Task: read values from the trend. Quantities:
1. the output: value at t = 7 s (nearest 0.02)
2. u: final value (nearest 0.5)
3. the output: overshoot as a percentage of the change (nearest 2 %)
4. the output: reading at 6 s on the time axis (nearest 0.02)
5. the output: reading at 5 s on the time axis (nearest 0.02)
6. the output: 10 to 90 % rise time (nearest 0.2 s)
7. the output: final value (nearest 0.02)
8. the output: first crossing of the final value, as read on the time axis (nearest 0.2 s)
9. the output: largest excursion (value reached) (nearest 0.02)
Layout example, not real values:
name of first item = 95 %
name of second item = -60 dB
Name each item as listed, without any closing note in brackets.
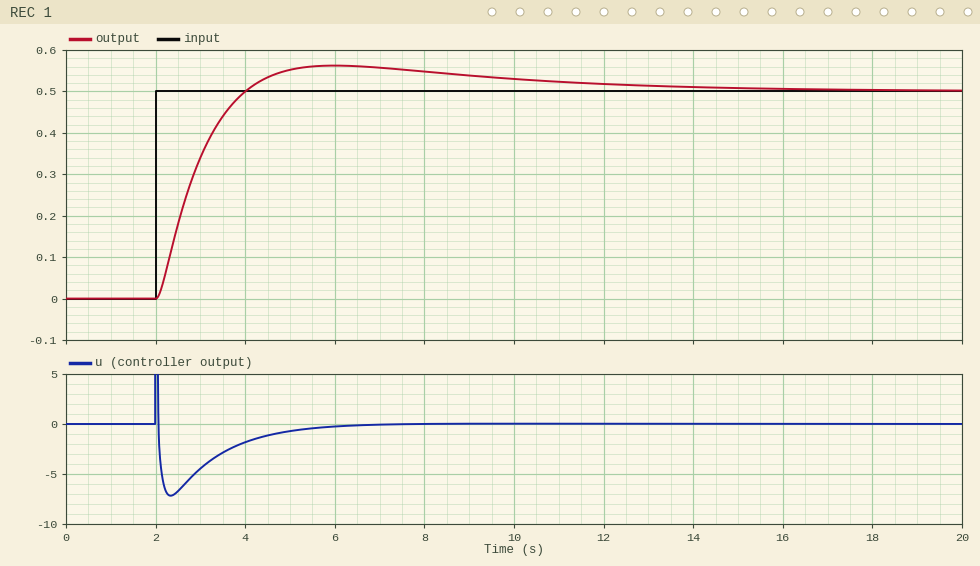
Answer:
the output: value at t = 7 s = 0.56
u: final value = 0.0
the output: overshoot as a percentage of the change = 12 %
the output: reading at 6 s on the time axis = 0.56
the output: reading at 5 s on the time axis = 0.56
the output: 10 to 90 % rise time = 1.4 s
the output: final value = 0.50
the output: first crossing of the final value, as read on the time axis = 4.0 s
the output: largest excursion (value reached) = 0.56
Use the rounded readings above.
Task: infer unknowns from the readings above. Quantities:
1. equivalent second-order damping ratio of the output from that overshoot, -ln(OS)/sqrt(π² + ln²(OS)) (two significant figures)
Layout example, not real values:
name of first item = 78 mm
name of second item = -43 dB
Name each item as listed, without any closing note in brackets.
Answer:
equivalent second-order damping ratio of the output from that overshoot, -ln(OS)/sqrt(π² + ln²(OS)) = 0.56
